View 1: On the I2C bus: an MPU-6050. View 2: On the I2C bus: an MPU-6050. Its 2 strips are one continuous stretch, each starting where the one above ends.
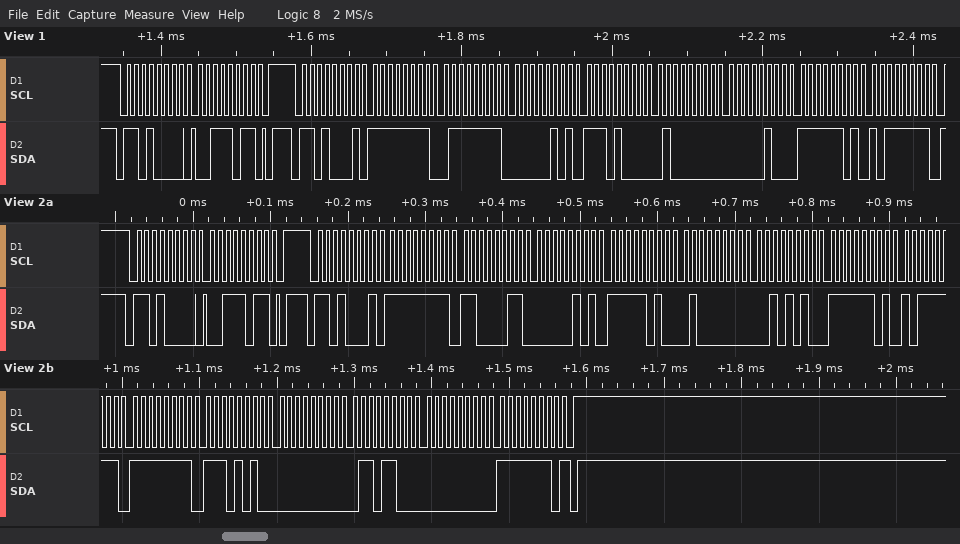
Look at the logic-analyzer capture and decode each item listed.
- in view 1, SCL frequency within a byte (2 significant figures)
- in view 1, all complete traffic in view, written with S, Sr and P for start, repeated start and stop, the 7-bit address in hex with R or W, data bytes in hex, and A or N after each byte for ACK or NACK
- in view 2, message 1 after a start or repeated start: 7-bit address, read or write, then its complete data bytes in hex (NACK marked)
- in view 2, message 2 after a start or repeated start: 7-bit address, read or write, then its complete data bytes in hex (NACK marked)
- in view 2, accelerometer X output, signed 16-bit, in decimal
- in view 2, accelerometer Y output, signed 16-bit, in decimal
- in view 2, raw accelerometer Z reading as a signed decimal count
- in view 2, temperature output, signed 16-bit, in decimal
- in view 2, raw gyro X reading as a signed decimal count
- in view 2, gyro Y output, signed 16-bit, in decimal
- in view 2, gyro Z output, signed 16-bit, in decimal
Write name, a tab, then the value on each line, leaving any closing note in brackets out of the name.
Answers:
in view 1, SCL frequency within a byte	100 kHz
in view 1, all complete traffic in view, written with S, Sr and P for start, repeated start and stop, the 7-bit address in hex with R or W, data bytes in hex, and A or N after each byte for ACK or NACK	S 68W A 3B A P S 68R A FF A 7F A 05 A E8 A 40 A 04 A FD A BF A
in view 2, message 1 after a start or repeated start: 7-bit address, read or write, then its complete data bytes in hex	0x68 write: 3B
in view 2, message 2 after a start or repeated start: 7-bit address, read or write, then its complete data bytes in hex	0x68 read: FF C3 05 FA 40 2A FD BF FF EA 00 6C 00 FE NACK
in view 2, accelerometer X output, signed 16-bit, in decimal	-61
in view 2, accelerometer Y output, signed 16-bit, in decimal	1530
in view 2, raw accelerometer Z reading as a signed decimal count	16426
in view 2, temperature output, signed 16-bit, in decimal	-577
in view 2, raw gyro X reading as a signed decimal count	-22
in view 2, gyro Y output, signed 16-bit, in decimal	108
in view 2, gyro Z output, signed 16-bit, in decimal	254
